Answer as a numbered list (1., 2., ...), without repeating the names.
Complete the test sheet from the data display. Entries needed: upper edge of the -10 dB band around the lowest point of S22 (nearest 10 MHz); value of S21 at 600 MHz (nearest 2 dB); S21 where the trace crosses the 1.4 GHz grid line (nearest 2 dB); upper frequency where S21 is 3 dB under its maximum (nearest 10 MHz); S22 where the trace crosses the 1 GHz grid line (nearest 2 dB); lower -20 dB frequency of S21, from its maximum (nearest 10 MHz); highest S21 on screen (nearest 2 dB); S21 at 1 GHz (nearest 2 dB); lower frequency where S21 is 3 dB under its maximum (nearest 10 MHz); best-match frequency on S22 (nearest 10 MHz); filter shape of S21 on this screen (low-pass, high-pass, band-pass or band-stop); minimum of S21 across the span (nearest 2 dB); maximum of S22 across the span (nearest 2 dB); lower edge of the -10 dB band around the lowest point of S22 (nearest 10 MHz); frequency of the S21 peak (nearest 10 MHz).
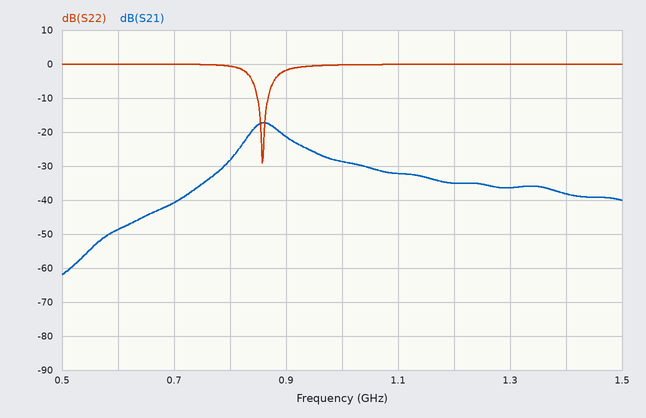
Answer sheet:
1. 870 MHz
2. -48 dB
3. -38 dB
4. 890 MHz
5. 0 dB
6. 730 MHz
7. -18 dB
8. -28 dB
9. 840 MHz
10. 860 MHz
11. band-pass
12. -62 dB
13. 0 dB
14. 850 MHz
15. 860 MHz
